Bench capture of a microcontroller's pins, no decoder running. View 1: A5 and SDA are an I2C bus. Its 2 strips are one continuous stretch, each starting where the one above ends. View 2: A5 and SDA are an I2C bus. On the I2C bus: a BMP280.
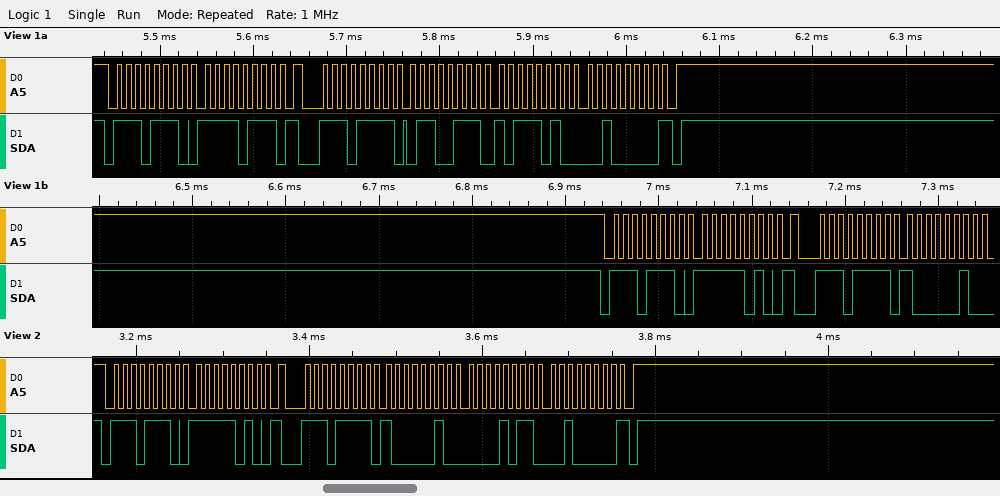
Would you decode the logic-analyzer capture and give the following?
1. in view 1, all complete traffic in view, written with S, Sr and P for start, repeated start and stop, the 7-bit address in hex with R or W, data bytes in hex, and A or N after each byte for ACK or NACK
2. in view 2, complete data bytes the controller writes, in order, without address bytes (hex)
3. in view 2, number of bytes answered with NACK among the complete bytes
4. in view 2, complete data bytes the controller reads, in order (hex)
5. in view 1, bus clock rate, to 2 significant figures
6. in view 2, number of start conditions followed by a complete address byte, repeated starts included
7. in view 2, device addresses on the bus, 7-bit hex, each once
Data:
S 77W A F7 A Sr 77R A 67 A BA A 20 N P S 77W A FA A Sr 77R A 82 A
FA
1
82 0B 20
100 kHz
2
0x77
